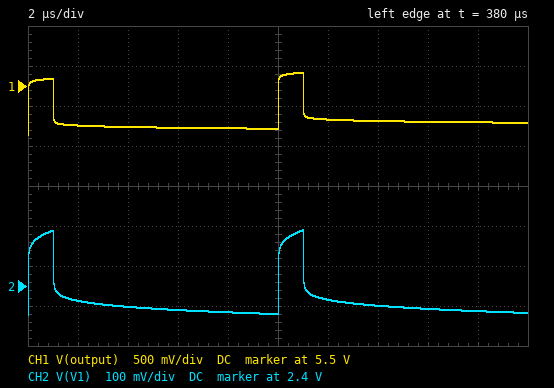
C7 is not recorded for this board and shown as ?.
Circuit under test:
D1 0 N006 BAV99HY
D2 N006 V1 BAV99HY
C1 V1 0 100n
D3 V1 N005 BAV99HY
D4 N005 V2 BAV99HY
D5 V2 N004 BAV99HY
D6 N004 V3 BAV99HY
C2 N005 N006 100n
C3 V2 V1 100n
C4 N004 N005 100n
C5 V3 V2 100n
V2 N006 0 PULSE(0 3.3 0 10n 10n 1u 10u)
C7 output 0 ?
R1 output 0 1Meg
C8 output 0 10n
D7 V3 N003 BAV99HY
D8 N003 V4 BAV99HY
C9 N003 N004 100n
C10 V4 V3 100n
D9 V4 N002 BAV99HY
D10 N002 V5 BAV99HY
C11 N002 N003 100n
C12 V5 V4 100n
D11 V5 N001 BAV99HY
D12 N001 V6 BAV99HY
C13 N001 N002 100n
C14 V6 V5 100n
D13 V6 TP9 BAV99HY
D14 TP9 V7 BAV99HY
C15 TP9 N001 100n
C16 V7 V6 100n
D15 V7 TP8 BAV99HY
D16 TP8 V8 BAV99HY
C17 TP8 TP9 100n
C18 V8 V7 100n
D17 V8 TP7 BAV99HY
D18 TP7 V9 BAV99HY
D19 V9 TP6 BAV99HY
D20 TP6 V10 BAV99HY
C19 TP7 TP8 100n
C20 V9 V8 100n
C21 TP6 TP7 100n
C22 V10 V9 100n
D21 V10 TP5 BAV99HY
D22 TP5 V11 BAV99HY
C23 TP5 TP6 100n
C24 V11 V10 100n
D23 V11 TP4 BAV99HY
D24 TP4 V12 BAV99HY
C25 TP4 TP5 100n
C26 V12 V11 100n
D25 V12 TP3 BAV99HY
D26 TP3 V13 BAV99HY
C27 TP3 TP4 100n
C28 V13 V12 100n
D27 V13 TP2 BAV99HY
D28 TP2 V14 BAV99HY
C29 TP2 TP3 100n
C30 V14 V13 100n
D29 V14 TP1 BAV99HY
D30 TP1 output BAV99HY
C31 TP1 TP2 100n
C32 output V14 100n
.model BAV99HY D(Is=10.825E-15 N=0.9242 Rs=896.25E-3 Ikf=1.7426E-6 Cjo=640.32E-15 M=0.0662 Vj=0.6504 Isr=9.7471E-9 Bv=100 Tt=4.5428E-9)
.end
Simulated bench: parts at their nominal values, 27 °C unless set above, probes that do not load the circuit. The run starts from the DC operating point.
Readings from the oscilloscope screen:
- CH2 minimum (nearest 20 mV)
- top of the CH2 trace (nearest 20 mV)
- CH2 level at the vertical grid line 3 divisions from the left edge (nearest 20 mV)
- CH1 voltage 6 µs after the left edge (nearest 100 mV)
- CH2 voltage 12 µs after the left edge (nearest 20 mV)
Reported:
2.32 V
2.54 V
2.34 V
5.0 V
2.36 V
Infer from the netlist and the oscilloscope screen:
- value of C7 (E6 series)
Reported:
3.3 nF
